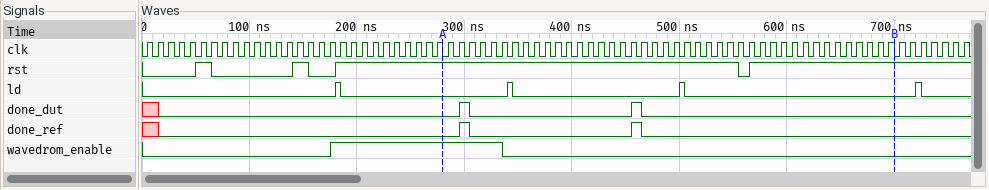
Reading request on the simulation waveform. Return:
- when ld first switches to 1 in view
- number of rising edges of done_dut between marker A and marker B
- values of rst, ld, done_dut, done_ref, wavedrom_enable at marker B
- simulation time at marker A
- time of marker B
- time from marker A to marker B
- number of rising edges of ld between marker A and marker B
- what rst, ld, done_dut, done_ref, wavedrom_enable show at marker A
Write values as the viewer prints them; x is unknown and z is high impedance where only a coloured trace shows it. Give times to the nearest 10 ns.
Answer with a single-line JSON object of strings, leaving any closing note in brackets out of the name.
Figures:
{"when ld first switches to 1 in view": "180 ns", "number of rising edges of done_dut between marker A and marker B": "2", "values of rst, ld, done_dut, done_ref, wavedrom_enable at marker B": "rst=1, ld=0, done_dut=0, done_ref=0, wavedrom_enable=0", "simulation time at marker A": "280 ns", "time of marker B": "700 ns", "time from marker A to marker B": "420 ns", "number of rising edges of ld between marker A and marker B": "2", "what rst, ld, done_dut, done_ref, wavedrom_enable show at marker A": "rst=1, ld=0, done_dut=0, done_ref=0, wavedrom_enable=1"}
